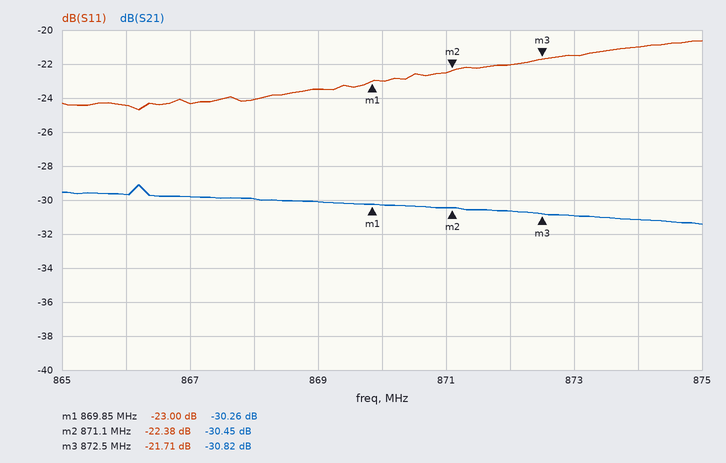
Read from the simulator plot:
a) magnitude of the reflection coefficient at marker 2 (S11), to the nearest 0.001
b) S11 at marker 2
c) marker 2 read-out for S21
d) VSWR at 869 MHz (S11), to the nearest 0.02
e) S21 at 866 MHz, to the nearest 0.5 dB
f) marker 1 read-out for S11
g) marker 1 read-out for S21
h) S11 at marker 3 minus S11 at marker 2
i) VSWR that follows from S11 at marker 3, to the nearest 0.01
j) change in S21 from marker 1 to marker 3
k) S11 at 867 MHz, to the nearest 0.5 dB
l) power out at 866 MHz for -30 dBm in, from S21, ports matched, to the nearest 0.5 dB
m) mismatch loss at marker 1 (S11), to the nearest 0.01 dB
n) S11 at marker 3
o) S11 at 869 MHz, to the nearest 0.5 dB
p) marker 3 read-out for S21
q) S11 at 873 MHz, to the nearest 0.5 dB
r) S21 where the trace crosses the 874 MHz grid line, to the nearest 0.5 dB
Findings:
0.076
-22.38 dB
-30.45 dB
1.14
-29.5 dB
-23.00 dB
-30.26 dB
0.67 dB
1.18
-0.56 dB
-24.5 dB
-59.5 dBm
0.02 dB
-21.71 dB
-23.5 dB
-30.82 dB
-21.5 dB
-31.0 dB
